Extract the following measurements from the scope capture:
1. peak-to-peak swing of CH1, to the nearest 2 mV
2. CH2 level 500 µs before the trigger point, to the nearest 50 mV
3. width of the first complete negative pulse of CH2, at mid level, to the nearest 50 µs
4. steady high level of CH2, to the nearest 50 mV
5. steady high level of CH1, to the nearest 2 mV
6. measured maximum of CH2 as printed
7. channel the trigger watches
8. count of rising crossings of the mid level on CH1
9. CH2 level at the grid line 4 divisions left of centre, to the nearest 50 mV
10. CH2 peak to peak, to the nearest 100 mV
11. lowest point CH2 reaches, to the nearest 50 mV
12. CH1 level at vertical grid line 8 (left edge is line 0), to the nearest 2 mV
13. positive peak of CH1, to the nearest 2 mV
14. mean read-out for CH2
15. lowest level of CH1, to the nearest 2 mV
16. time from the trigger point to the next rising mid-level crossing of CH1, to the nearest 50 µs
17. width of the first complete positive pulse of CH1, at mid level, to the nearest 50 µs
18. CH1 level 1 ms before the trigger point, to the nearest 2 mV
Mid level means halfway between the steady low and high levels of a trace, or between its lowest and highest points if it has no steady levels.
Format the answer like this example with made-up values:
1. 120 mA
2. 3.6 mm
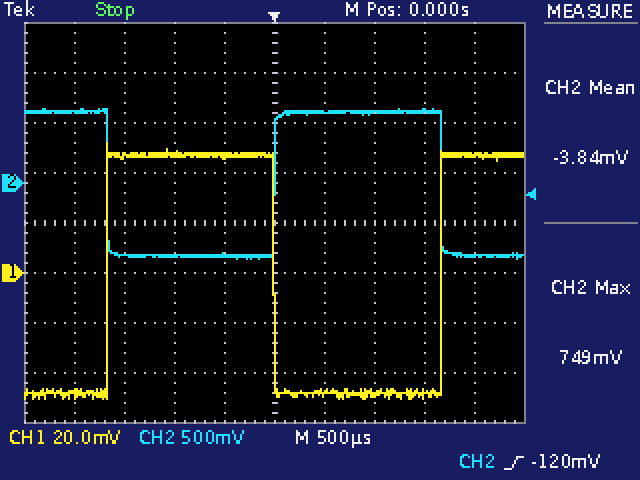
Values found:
1. 102 mV
2. -700 mV
3. 1.65 ms
4. 700 mV
5. 48 mV
6. 749 mV
7. CH2
8. 2
9. 700 mV
10. 1.50 V
11. -750 mV
12. -48 mV
13. 52 mV
14. -3.84 mV
15. -50 mV
16. 1.65 ms
17. 1.65 ms
18. 48 mV
